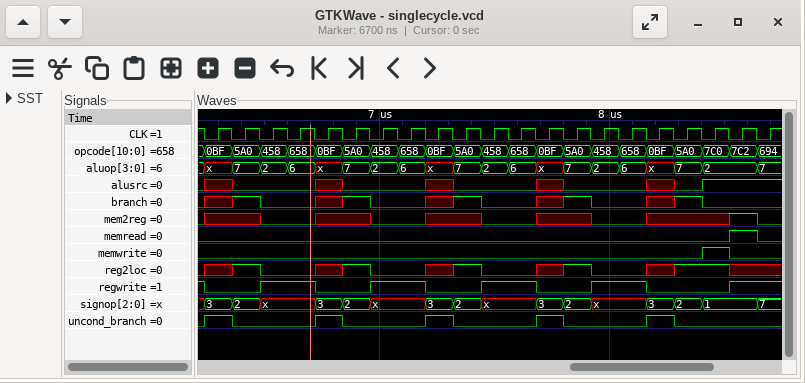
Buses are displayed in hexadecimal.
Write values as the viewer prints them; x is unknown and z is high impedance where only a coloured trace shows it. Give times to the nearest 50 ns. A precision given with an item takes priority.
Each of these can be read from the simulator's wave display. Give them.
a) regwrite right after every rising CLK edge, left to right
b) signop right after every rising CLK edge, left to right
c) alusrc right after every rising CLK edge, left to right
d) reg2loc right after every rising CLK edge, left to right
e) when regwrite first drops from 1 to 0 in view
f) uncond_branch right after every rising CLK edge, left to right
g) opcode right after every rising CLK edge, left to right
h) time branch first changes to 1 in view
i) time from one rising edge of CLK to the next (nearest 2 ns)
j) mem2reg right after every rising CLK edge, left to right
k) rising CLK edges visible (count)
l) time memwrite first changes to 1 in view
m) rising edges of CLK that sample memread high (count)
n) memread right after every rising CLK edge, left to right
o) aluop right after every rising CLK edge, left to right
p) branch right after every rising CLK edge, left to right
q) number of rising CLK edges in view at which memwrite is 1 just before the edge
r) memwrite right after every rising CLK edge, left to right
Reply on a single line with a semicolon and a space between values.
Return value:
0 0 1 1 0 0 1 1 0 0 1 1 0 0 1 1 0 0 0 1 1; 3, 2, x, x, 3, 2, x, x, 3, 2, x, x, 3, 2, x, x, 3, 2, 1, 1, 7; x 0 0 0 x 0 0 0 x 0 0 0 x 0 0 0 x 0 1 1 1; x 1 0 0 x 1 0 0 x 1 0 0 x 1 0 0 x 1 1 x x; 6250 ns; 1 0 0 0 1 0 0 0 1 0 0 0 1 0 0 0 1 0 0 0 0; 0BF, 5A0, 458, 658, 0BF, 5A0, 458, 658, 0BF, 5A0, 458, 658, 0BF, 5A0, 458, 658, 0BF, 5A0, 7C0, 7C2, 694; 6350 ns; 120 ns; x x 0 0 x x 0 0 x x 0 0 x x 0 0 x x x 1 0; 21; 8400 ns; 1; 0 0 0 0 0 0 0 0 0 0 0 0 0 0 0 0 0 0 0 1 0; x, 7, 2, 6, x, 7, 2, 6, x, 7, 2, 6, x, 7, 2, 6, x, 7, 2, 2, 7; x 1 0 0 x 1 0 0 x 1 0 0 x 1 0 0 x 1 0 0 0; 1; 0 0 0 0 0 0 0 0 0 0 0 0 0 0 0 0 0 0 1 0 0
